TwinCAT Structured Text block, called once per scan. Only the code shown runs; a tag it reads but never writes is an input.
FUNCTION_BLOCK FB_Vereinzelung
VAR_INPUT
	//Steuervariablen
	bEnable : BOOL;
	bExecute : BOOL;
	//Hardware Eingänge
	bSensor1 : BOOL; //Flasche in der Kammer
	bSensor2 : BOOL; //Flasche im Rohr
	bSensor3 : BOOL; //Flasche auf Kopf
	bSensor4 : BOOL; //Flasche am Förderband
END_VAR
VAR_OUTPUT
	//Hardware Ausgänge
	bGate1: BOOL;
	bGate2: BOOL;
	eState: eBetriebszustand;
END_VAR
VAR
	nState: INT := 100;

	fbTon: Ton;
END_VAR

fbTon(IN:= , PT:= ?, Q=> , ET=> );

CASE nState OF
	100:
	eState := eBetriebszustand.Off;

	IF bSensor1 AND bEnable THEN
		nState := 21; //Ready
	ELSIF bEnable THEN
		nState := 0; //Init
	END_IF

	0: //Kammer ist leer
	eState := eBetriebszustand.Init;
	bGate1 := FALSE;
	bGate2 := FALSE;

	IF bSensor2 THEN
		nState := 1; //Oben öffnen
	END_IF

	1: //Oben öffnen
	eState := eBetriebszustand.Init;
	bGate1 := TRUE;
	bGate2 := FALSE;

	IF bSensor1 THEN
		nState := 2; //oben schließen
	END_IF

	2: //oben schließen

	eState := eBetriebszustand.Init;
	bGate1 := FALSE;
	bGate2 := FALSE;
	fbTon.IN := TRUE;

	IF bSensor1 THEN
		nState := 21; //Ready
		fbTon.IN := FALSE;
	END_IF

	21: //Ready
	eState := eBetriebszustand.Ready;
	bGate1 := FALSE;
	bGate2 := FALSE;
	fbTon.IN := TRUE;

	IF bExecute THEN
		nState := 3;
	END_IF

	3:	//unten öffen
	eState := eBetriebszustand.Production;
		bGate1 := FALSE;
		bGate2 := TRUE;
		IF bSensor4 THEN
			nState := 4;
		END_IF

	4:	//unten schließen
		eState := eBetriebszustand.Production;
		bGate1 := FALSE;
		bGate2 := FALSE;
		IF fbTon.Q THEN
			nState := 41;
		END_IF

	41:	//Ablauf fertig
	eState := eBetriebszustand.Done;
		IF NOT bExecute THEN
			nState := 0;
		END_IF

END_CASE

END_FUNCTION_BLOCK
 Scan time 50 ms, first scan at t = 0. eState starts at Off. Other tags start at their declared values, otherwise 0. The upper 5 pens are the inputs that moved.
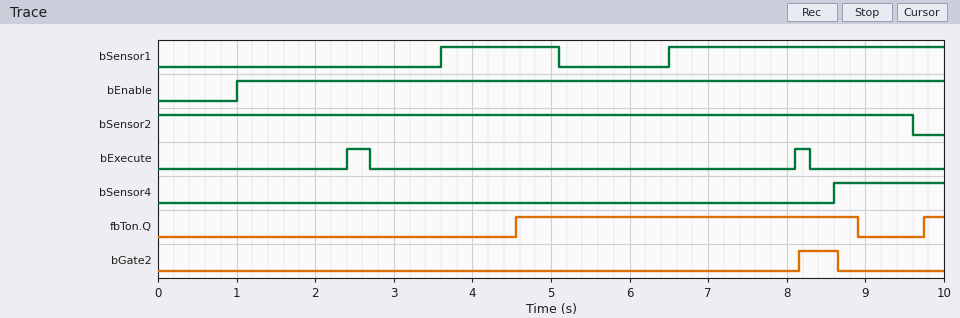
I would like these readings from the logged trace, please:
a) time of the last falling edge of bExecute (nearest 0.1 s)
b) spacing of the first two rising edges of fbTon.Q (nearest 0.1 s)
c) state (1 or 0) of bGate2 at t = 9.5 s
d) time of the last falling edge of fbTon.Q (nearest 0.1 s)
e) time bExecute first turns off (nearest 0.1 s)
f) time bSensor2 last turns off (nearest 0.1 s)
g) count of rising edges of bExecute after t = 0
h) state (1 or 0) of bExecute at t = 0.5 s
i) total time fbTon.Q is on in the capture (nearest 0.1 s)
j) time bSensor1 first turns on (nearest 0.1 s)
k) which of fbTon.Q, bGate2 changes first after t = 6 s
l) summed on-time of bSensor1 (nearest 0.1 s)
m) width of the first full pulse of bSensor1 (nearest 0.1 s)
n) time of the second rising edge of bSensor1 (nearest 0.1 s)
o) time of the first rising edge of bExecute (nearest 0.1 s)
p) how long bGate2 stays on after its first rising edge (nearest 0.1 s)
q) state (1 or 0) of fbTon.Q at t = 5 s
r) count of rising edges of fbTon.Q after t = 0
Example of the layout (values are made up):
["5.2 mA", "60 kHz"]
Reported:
["8.3 s", "5.2 s", "0", "8.9 s", "2.7 s", "9.6 s", "2", "0", "4.6 s", "3.6 s", "bGate2", "5.0 s", "1.5 s", "6.5 s", "2.4 s", "0.5 s", "1", "2"]
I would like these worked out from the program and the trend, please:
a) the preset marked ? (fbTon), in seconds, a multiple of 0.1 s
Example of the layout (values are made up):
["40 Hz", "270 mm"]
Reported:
["0.8 s"]
